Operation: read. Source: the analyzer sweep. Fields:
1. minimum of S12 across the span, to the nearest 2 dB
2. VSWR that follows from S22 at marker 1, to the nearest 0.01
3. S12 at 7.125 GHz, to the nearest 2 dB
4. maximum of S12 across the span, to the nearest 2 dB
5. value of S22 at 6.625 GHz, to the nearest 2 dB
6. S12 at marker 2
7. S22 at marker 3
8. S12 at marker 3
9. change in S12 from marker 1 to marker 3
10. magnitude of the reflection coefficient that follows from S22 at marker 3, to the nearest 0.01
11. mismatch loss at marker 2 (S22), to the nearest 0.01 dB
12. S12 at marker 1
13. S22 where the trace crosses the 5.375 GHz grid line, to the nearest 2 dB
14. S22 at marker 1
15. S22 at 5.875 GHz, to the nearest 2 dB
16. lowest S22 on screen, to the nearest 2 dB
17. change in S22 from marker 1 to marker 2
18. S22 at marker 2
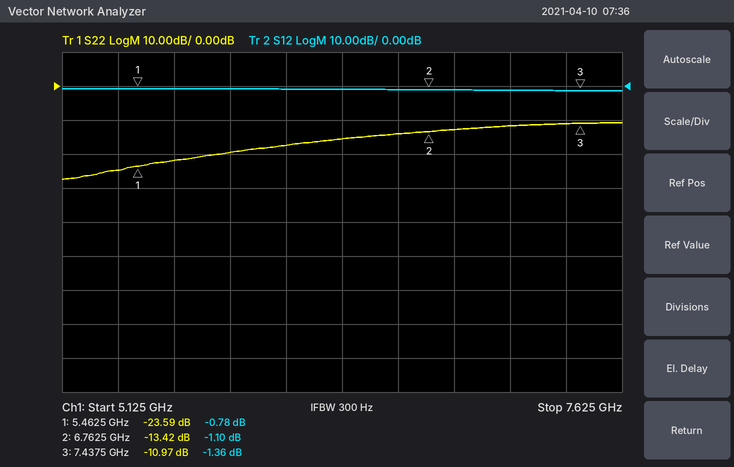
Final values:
-2 dB
1.14
-2 dB
0 dB
-14 dB
-1.10 dB
-10.97 dB
-1.36 dB
-0.58 dB
0.28
0.20 dB
-0.78 dB
-24 dB
-23.59 dB
-20 dB
-28 dB
10.17 dB
-13.42 dB
